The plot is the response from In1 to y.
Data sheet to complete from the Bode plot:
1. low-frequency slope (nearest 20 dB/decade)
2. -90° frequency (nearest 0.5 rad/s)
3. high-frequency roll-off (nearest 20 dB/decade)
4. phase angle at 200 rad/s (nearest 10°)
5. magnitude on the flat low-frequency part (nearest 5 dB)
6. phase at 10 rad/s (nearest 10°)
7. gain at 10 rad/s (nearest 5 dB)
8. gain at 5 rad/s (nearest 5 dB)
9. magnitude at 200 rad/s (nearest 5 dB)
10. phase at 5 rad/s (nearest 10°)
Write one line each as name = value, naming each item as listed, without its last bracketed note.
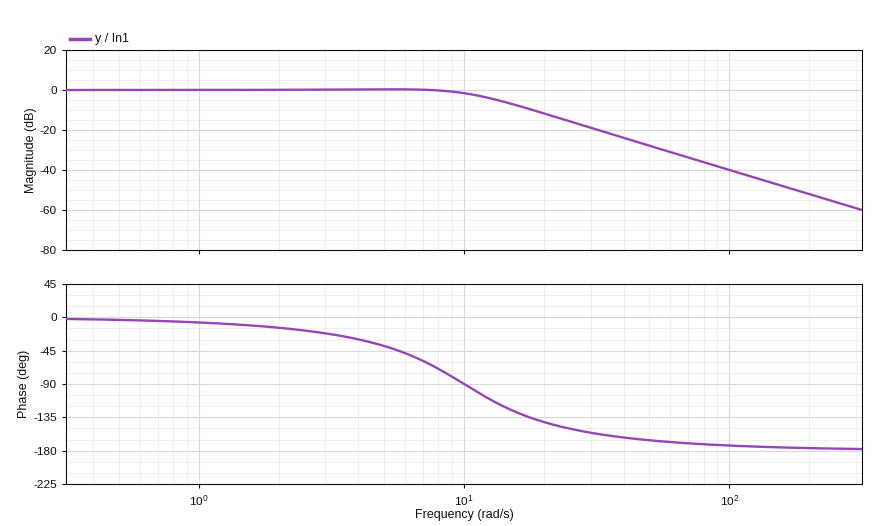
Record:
low-frequency slope = 0 dB/decade
-90° frequency = 10.0 rad/s
high-frequency roll-off = -40 dB/decade
phase angle at 200 rad/s = -180°
magnitude on the flat low-frequency part = 0 dB
phase at 10 rad/s = -90°
gain at 10 rad/s = 0 dB
gain at 5 rad/s = 0 dB
magnitude at 200 rad/s = -50 dB
phase at 5 rad/s = -40°
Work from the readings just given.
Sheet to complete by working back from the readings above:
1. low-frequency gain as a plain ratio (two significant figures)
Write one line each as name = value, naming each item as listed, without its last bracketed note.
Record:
low-frequency gain as a plain ratio = 1.0
